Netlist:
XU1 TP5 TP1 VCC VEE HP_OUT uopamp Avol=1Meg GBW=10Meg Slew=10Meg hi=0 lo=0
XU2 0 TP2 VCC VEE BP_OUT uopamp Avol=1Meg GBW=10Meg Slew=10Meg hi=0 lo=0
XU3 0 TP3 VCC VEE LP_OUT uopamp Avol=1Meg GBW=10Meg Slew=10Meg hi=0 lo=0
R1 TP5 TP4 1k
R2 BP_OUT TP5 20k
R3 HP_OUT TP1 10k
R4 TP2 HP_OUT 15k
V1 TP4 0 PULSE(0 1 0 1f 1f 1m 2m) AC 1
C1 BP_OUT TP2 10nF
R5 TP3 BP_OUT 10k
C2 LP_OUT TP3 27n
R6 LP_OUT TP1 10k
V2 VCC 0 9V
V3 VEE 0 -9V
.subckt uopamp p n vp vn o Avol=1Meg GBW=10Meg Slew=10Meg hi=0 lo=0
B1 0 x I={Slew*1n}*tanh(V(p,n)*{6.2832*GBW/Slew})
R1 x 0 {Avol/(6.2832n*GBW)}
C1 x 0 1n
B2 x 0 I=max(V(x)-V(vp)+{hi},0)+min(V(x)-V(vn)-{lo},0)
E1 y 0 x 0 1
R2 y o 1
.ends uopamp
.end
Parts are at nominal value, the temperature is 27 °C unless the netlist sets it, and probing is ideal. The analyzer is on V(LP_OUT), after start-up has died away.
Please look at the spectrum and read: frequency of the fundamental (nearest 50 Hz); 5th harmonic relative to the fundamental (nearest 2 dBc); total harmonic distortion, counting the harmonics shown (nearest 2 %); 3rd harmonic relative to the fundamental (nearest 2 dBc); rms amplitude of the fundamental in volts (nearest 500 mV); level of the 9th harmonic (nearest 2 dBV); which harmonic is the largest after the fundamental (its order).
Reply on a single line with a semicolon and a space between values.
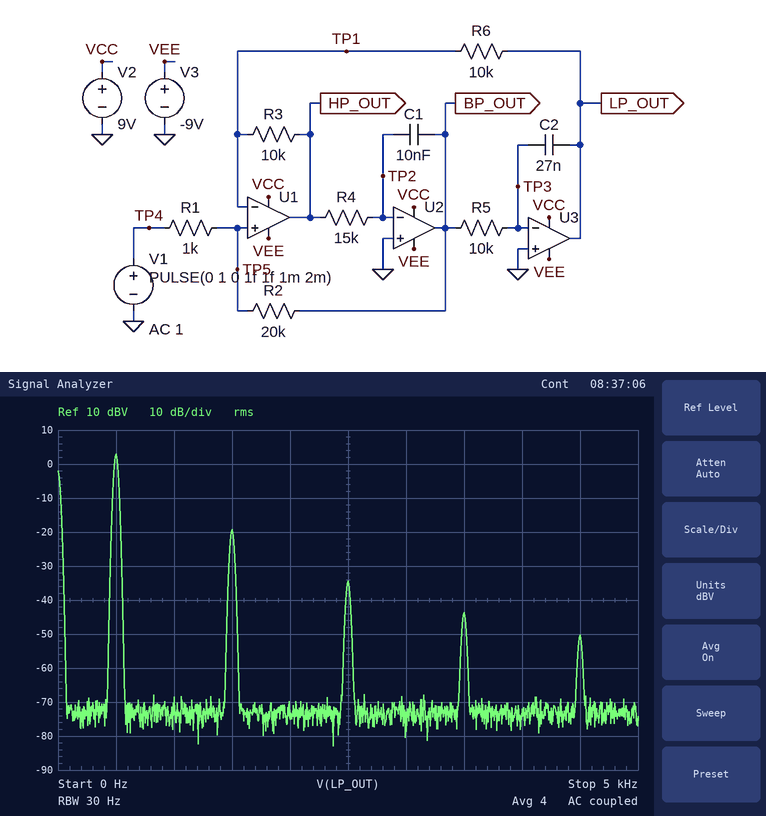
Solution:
500 Hz; -38 dBc; 8 %; -22 dBc; 1.5 V; -50 dBV; 3
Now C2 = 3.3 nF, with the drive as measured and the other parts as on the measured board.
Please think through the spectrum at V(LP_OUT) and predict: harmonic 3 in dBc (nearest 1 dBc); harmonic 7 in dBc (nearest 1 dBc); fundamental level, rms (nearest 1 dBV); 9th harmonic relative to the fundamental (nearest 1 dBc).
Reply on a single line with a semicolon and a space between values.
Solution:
-5 dBc; -20 dBc; -1 dBV; -29 dBc
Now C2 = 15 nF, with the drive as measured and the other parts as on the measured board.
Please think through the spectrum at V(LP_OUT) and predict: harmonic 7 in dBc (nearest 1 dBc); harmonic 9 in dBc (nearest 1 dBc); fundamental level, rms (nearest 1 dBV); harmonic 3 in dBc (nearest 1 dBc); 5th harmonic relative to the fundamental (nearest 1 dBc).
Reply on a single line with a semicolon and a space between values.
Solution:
-39 dBc; -46 dBc; 1 dBV; -12 dBc; -29 dBc
